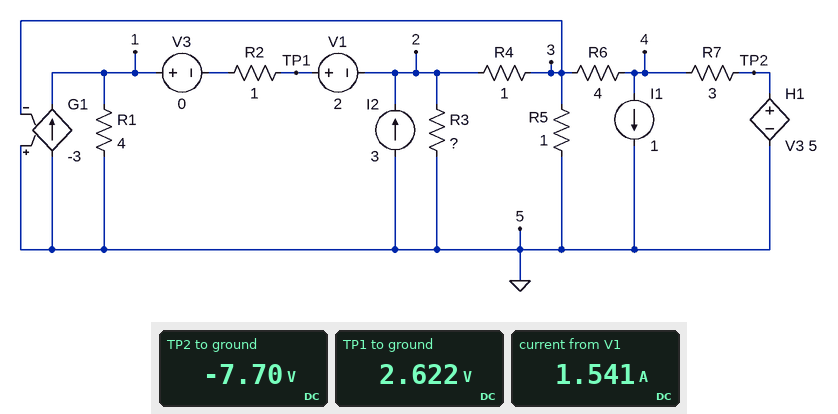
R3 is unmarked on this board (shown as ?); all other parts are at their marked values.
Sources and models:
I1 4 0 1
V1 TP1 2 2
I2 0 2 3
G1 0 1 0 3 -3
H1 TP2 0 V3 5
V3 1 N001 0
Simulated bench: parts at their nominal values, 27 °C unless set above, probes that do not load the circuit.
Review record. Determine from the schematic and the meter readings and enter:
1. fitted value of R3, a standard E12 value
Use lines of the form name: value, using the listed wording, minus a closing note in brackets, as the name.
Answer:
fitted value of R3, a standard E12 value: 1.5 Ω
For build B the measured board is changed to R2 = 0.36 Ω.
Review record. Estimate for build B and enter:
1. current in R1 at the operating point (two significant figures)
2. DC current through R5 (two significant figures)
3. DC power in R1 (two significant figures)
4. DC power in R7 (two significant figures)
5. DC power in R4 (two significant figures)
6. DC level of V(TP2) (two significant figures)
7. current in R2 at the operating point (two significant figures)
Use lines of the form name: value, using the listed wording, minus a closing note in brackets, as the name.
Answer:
current in R1 at the operating point: 590 mA
DC current through R5: 250 mA
DC power in R1: 1.4 W
DC power in R7: 360 mW
DC power in R4: 1.2 W
DC level of V(TP2): -6.7 V
current in R2 at the operating point: 1.3 A
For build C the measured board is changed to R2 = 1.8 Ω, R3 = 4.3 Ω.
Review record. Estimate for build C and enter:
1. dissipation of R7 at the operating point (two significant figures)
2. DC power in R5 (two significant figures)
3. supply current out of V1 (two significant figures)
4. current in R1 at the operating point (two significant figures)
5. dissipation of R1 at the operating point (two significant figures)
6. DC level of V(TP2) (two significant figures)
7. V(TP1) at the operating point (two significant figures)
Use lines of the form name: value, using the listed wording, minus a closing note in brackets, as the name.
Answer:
dissipation of R7 at the operating point: 1.7 W
DC power in R5: 620 mW
supply current out of V1: 2.0 A
current in R1 at the operating point: 360 mA
dissipation of R1 at the operating point: 510 mW
DC level of V(TP2): -10 V
V(TP1) at the operating point: 2.2 V
